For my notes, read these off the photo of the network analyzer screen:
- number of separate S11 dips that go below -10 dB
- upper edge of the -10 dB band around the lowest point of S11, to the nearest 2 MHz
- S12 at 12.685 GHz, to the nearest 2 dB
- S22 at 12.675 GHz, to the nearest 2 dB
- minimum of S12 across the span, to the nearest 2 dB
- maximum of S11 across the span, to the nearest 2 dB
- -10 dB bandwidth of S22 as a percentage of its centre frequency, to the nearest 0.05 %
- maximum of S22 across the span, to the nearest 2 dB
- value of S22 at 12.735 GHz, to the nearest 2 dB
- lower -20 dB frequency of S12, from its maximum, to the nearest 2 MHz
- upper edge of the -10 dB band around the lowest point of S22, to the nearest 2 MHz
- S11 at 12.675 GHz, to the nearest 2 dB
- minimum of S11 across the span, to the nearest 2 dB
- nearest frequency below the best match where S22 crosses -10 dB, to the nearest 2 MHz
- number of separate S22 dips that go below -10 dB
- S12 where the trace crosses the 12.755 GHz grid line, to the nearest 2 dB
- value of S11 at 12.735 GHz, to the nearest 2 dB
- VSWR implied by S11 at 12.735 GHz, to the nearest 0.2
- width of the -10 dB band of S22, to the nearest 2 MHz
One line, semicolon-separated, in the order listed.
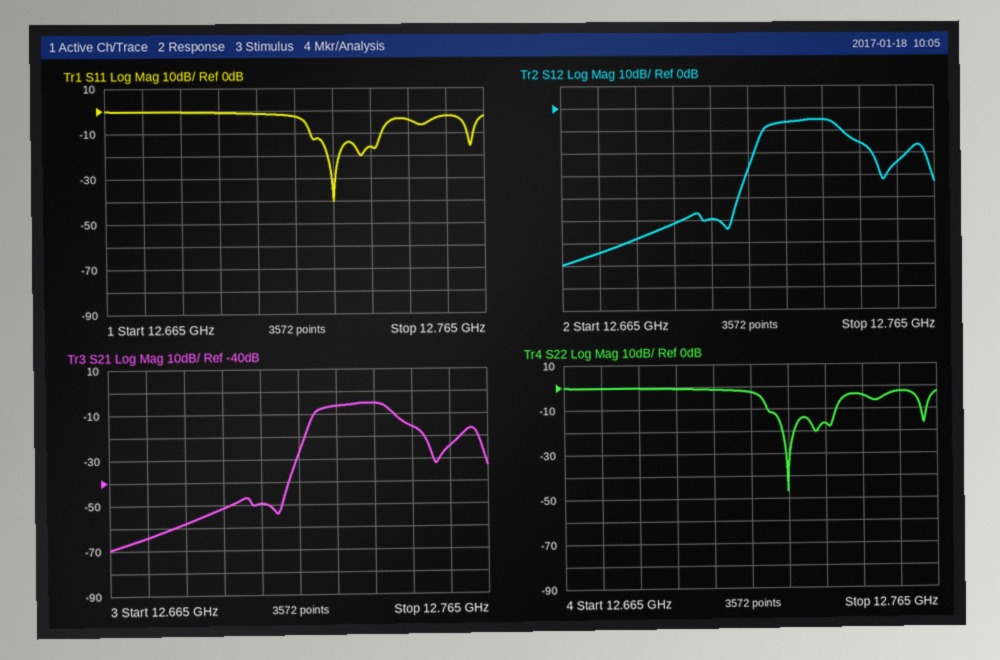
3; 12.738 GHz; -58 dB; 0 dB; -70 dB; 0 dB; 0.15 %; 0 dB; -16 dB; 12.716 GHz; 12.738 GHz; 0 dB; -40 dB; 12.720 GHz; 3; -24 dB; -16 dB; 1.4; 18 MHz
